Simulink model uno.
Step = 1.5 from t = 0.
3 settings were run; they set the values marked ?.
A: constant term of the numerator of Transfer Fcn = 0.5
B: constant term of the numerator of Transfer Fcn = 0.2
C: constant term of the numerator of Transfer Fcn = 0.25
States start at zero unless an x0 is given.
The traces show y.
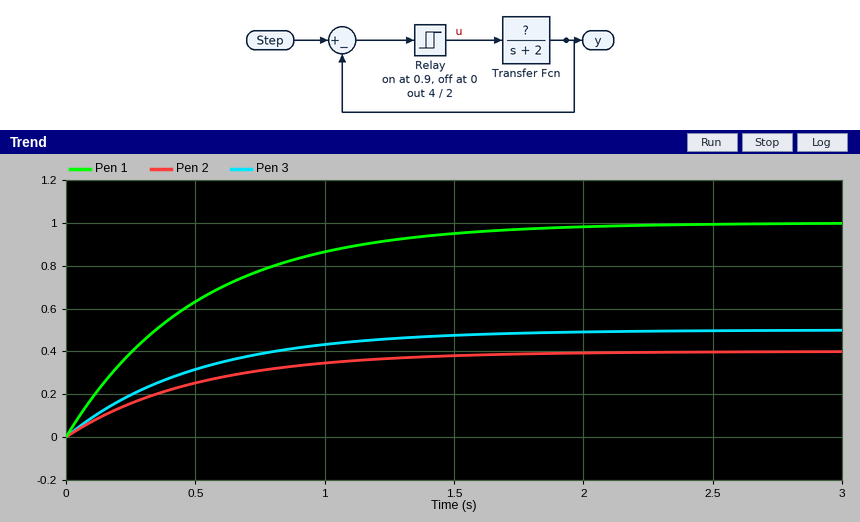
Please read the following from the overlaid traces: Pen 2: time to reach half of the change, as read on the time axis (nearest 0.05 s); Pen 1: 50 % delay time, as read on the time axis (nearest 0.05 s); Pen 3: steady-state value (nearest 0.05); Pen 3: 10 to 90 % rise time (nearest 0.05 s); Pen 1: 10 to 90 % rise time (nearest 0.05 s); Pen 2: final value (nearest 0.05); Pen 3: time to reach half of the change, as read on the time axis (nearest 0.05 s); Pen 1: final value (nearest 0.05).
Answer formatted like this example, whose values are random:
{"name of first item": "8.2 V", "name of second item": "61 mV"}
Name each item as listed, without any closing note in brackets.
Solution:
{"Pen 2: time to reach half of the change, as read on the time axis": "0.35 s", "Pen 1: 50 % delay time, as read on the time axis": "0.35 s", "Pen 3: steady-state value": "0.50", "Pen 3: 10 to 90 % rise time": "1.10 s", "Pen 1: 10 to 90 % rise time": "1.10 s", "Pen 2: final value": "0.40", "Pen 3: time to reach half of the change, as read on the time axis": "0.35 s", "Pen 1: final value": "1.00"}
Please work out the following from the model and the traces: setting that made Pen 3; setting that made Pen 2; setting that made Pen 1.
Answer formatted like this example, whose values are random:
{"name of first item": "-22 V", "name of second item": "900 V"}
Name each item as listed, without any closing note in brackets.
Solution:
{"setting that made Pen 3": "C", "setting that made Pen 2": "B", "setting that made Pen 1": "A"}
